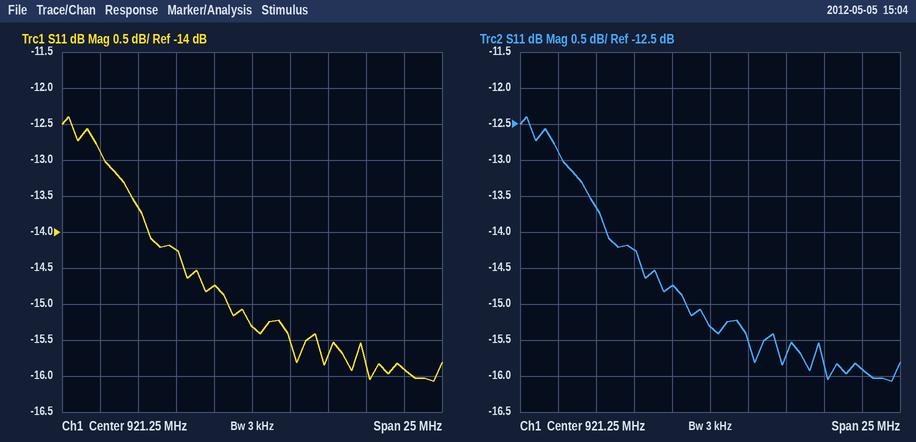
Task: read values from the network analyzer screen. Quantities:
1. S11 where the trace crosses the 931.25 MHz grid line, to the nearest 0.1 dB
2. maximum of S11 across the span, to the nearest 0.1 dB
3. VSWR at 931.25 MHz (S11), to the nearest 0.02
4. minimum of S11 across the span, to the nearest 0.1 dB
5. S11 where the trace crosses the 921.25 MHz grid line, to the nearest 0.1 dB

-15.9 dB
-12.4 dB
1.38
-16.1 dB
-15.3 dB
